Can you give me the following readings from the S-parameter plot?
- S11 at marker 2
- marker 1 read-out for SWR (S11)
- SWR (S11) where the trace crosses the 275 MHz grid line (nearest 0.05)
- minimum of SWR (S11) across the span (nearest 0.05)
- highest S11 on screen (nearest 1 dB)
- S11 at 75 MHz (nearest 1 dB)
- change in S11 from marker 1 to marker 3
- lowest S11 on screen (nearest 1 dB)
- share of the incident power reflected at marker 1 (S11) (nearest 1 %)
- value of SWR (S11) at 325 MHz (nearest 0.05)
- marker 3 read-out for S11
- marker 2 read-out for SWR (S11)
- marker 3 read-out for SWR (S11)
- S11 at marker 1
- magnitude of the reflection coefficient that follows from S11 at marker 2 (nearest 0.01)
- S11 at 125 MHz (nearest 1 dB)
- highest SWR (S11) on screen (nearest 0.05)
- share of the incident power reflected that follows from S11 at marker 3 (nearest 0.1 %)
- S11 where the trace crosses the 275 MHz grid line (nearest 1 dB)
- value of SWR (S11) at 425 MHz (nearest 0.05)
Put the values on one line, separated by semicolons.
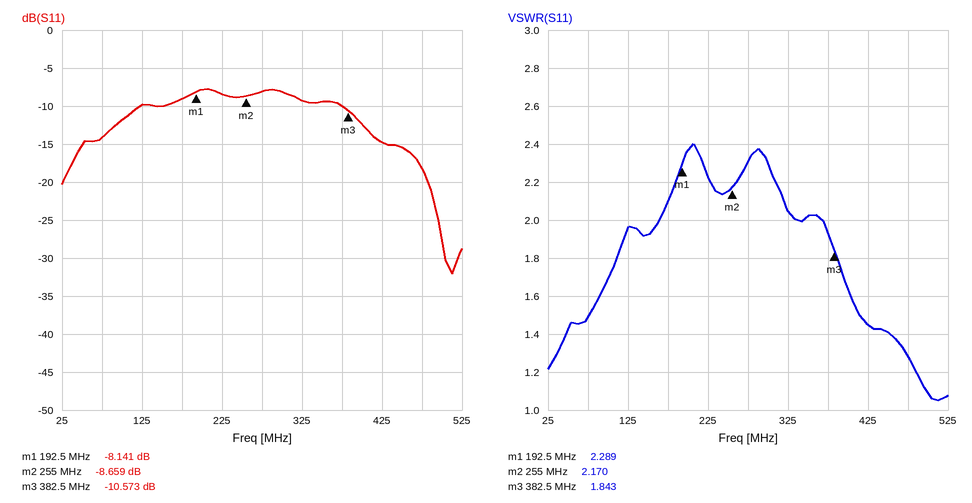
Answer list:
-8.659 dB; 2.289; 2.30; 1.05; -8 dB; -14 dB; -2.432 dB; -32 dB; 15 %; 2.05; -10.573 dB; 2.170; 1.843; -8.141 dB; 0.37; -10 dB; 2.40; 8.8 %; -8 dB; 1.45
